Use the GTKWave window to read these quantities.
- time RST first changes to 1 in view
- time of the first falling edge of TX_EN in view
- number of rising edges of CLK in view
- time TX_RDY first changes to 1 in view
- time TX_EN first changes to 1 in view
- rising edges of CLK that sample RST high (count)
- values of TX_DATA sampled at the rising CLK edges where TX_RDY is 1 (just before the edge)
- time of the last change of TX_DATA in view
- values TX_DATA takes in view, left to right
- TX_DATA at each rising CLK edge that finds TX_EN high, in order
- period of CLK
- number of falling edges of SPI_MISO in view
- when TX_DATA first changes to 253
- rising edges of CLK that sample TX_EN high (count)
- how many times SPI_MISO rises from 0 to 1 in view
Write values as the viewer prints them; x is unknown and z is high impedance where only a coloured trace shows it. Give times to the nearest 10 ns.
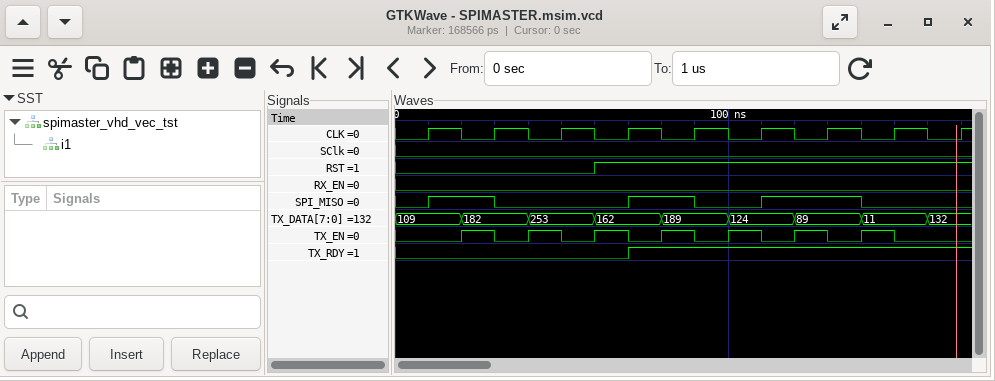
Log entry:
60 ns
30 ns
9
70 ns
20 ns
6
189, 124, 89, 11, 132
160 ns
109, 182, 253, 162, 189, 124, 89, 11, 132
182, 253, 162, 189, 124, 89, 11
20 ns
3
40 ns
7
3
